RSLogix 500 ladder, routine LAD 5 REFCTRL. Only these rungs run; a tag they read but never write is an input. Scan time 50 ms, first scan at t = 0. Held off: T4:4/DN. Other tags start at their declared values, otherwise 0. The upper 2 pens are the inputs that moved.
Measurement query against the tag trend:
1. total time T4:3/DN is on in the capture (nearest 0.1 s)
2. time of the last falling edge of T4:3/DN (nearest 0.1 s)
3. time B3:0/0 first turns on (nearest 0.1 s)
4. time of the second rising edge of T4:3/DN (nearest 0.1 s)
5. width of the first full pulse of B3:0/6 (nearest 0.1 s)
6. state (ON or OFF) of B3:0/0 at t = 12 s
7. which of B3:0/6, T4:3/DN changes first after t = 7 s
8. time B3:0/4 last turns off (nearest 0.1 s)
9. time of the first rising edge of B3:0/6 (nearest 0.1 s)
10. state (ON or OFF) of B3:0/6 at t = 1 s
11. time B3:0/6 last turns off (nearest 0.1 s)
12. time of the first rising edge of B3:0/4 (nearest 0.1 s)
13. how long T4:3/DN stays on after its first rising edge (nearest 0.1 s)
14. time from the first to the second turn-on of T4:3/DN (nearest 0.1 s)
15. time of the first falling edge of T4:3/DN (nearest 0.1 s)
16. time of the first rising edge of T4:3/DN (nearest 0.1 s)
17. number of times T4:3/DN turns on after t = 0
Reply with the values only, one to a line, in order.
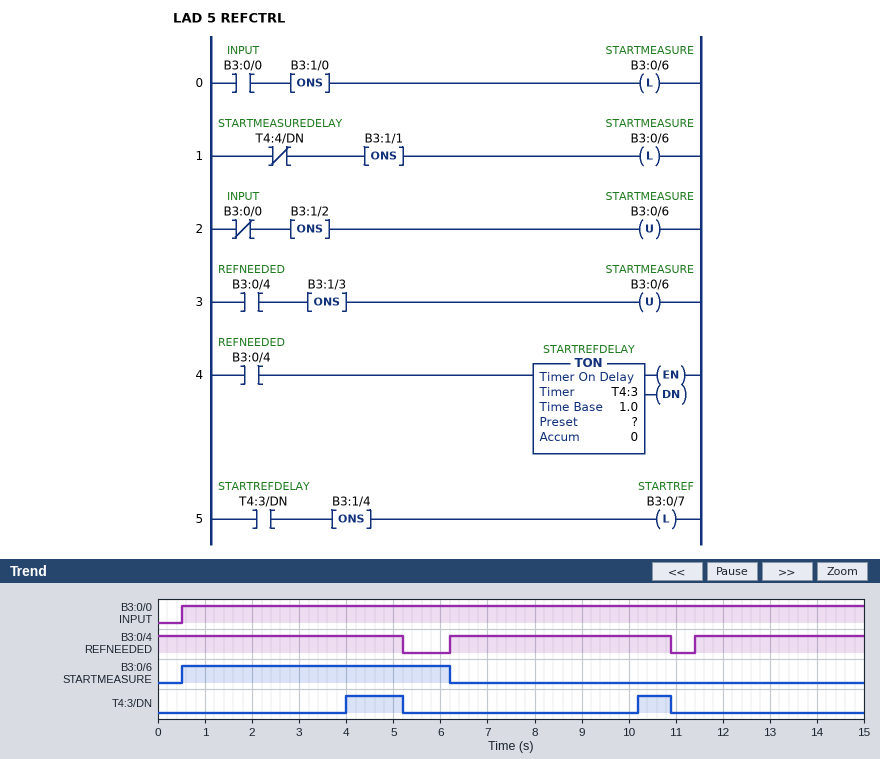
1.9 s
10.9 s
0.5 s
10.2 s
5.7 s
ON
T4:3/DN
10.9 s
0.5 s
ON
6.2 s
6.2 s
1.2 s
6.2 s
5.2 s
4.0 s
2
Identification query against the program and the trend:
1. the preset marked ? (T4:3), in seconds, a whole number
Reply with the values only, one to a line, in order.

4 s
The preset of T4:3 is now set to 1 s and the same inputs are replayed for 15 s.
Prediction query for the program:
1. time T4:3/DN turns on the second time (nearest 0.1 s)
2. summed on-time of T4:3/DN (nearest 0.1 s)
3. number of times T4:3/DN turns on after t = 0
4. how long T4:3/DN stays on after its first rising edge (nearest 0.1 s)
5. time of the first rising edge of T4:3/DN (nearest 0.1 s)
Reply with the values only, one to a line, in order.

7.2 s
10.5 s
3
4.2 s
1.0 s
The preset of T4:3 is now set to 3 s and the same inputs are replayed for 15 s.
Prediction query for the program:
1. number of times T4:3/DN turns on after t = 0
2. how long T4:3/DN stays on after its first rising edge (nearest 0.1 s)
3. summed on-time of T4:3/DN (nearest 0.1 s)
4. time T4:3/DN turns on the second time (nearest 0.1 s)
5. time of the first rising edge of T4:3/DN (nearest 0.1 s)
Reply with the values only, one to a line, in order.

3
2.2 s
4.5 s
9.2 s
3.0 s
